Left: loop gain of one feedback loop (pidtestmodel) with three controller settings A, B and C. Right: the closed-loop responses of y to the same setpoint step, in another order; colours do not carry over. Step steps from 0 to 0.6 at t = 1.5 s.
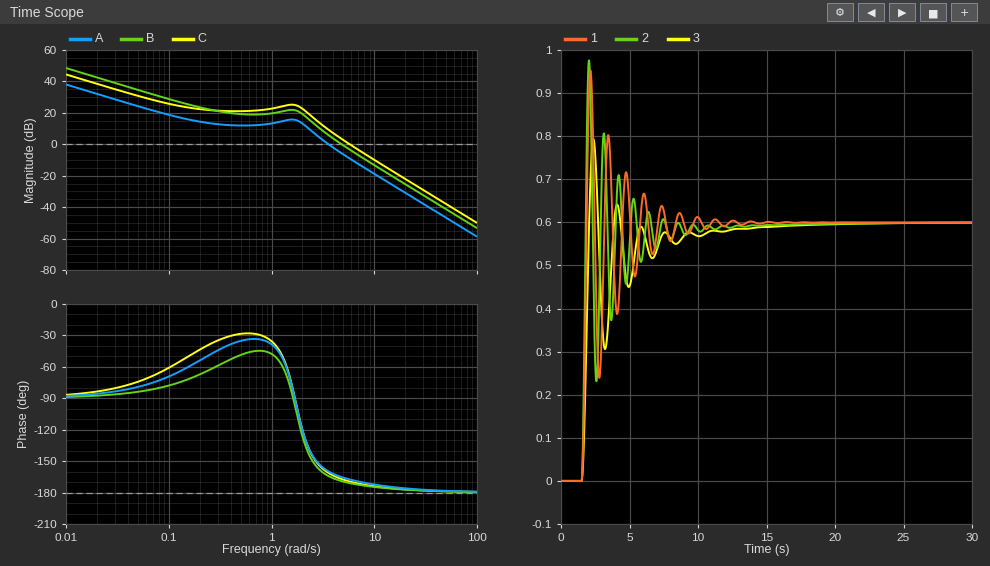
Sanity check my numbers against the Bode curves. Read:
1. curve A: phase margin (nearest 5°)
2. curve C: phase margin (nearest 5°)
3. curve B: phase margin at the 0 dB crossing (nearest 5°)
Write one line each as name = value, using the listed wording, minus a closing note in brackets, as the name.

curve A: phase margin = 20°
curve C: phase margin = 10°
curve B: phase margin at the 0 dB crossing = 10°
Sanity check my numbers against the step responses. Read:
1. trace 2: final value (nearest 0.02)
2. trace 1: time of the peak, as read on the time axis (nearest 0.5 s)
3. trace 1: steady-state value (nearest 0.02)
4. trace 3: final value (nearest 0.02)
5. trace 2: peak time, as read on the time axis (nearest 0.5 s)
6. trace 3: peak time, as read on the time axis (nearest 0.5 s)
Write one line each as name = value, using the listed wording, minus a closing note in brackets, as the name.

trace 2: final value = 0.60
trace 1: time of the peak, as read on the time axis = 2.0 s
trace 1: steady-state value = 0.60
trace 3: final value = 0.60
trace 2: peak time, as read on the time axis = 2.0 s
trace 3: peak time, as read on the time axis = 2.5 s
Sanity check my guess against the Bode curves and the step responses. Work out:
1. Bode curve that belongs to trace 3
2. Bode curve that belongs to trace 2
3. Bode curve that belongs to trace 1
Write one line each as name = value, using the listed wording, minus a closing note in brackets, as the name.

Bode curve that belongs to trace 3 = A
Bode curve that belongs to trace 2 = C
Bode curve that belongs to trace 1 = B
